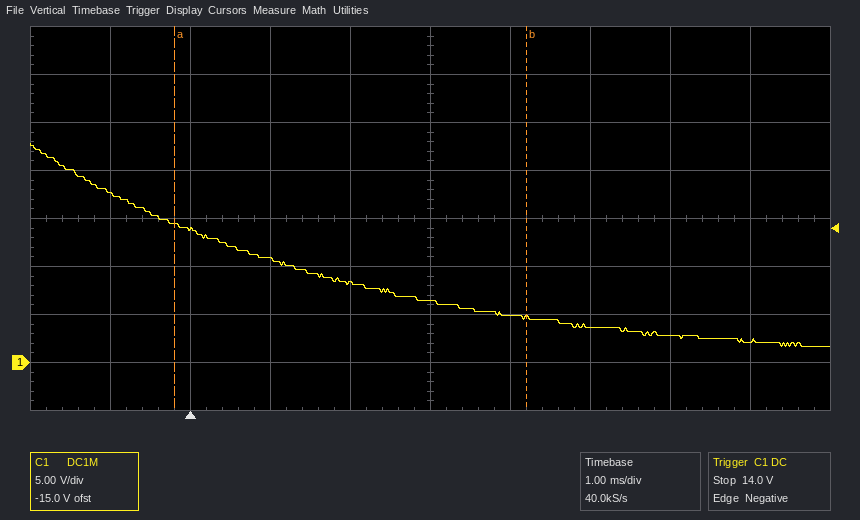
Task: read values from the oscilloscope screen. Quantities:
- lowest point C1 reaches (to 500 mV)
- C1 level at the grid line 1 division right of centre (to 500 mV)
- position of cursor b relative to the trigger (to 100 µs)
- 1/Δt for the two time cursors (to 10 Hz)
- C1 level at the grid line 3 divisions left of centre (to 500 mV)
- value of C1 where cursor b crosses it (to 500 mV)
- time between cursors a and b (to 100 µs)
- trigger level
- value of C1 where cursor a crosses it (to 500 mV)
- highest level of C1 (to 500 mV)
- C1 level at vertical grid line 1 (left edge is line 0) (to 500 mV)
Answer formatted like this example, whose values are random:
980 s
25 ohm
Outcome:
1.5 V
5.0 V
+4.2 ms
230 Hz
14.0 V
4.5 V
4.4 ms
14.0 V
14.5 V
23.0 V
17.5 V
